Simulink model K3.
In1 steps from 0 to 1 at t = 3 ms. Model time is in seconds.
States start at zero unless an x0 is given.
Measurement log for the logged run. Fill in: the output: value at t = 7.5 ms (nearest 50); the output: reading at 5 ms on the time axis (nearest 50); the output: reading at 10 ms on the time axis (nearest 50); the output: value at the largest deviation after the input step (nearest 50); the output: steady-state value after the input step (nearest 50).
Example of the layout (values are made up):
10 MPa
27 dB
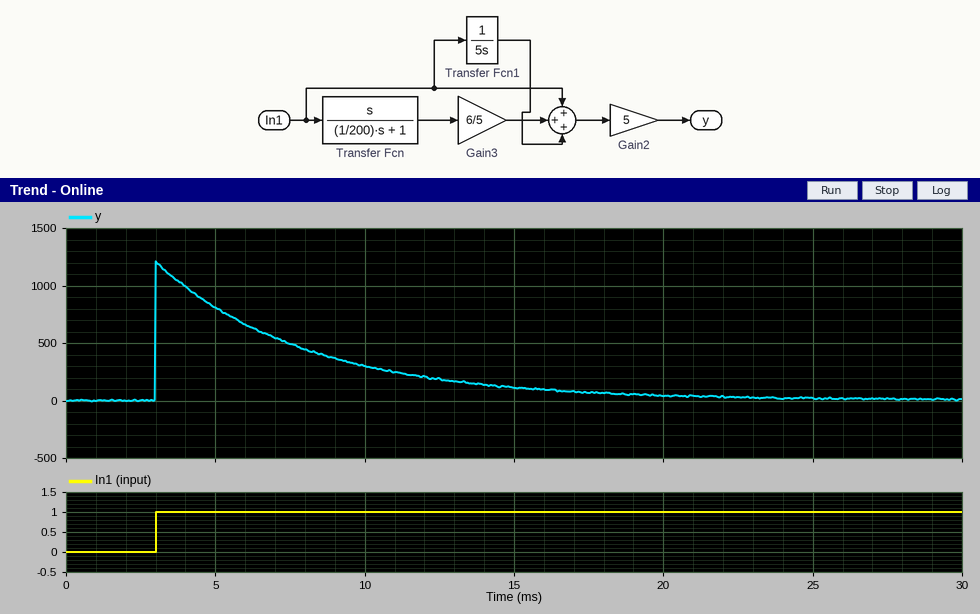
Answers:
500
800
300
1200
0
